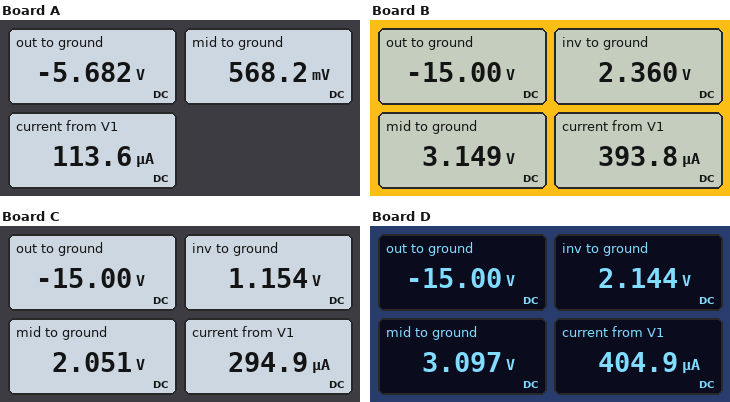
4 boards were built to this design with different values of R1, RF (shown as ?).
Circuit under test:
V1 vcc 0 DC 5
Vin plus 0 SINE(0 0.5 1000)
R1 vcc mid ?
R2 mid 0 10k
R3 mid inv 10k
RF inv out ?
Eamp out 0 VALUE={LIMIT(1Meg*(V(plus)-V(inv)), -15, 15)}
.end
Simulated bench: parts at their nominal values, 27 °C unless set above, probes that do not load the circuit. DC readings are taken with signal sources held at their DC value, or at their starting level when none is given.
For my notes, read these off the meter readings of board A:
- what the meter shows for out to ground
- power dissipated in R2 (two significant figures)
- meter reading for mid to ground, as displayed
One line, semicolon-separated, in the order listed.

-5.682 V; 32 µW; 568.2 mV
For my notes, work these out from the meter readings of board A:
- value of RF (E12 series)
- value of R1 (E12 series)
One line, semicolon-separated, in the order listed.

100 kΩ; 39 kΩ
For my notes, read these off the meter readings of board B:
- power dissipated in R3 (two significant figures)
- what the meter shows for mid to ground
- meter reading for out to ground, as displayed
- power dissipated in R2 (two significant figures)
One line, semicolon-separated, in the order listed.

62 µW; 3.149 V; -15.00 V; 990 µW
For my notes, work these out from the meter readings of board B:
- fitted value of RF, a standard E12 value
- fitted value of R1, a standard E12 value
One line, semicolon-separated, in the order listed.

220 kΩ; 4.7 kΩ
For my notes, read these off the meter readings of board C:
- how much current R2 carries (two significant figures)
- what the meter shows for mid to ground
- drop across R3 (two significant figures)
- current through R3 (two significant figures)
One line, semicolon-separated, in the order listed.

210 µA; 2.051 V; 900 mV; 90 µA
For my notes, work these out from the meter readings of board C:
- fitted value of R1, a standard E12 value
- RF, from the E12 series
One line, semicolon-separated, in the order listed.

10 kΩ; 180 kΩ
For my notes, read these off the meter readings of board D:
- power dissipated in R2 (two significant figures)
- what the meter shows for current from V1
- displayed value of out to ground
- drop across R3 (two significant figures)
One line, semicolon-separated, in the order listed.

960 µW; 404.9 µA; -15.00 V; 950 mV
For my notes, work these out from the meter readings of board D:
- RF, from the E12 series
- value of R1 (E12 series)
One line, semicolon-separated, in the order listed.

180 kΩ; 4.7 kΩ
